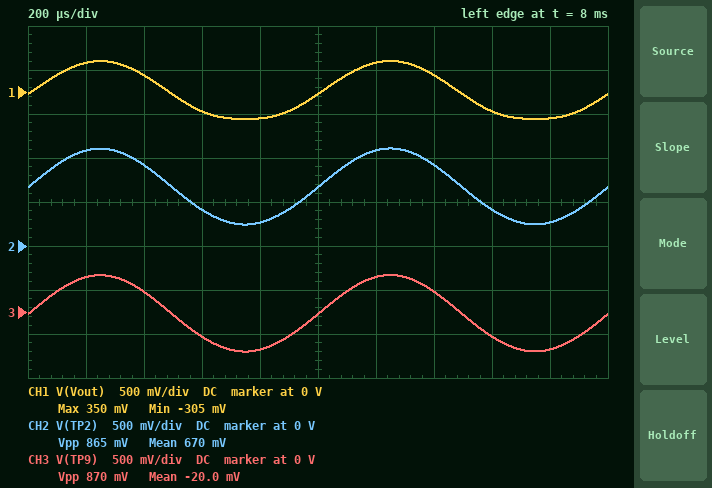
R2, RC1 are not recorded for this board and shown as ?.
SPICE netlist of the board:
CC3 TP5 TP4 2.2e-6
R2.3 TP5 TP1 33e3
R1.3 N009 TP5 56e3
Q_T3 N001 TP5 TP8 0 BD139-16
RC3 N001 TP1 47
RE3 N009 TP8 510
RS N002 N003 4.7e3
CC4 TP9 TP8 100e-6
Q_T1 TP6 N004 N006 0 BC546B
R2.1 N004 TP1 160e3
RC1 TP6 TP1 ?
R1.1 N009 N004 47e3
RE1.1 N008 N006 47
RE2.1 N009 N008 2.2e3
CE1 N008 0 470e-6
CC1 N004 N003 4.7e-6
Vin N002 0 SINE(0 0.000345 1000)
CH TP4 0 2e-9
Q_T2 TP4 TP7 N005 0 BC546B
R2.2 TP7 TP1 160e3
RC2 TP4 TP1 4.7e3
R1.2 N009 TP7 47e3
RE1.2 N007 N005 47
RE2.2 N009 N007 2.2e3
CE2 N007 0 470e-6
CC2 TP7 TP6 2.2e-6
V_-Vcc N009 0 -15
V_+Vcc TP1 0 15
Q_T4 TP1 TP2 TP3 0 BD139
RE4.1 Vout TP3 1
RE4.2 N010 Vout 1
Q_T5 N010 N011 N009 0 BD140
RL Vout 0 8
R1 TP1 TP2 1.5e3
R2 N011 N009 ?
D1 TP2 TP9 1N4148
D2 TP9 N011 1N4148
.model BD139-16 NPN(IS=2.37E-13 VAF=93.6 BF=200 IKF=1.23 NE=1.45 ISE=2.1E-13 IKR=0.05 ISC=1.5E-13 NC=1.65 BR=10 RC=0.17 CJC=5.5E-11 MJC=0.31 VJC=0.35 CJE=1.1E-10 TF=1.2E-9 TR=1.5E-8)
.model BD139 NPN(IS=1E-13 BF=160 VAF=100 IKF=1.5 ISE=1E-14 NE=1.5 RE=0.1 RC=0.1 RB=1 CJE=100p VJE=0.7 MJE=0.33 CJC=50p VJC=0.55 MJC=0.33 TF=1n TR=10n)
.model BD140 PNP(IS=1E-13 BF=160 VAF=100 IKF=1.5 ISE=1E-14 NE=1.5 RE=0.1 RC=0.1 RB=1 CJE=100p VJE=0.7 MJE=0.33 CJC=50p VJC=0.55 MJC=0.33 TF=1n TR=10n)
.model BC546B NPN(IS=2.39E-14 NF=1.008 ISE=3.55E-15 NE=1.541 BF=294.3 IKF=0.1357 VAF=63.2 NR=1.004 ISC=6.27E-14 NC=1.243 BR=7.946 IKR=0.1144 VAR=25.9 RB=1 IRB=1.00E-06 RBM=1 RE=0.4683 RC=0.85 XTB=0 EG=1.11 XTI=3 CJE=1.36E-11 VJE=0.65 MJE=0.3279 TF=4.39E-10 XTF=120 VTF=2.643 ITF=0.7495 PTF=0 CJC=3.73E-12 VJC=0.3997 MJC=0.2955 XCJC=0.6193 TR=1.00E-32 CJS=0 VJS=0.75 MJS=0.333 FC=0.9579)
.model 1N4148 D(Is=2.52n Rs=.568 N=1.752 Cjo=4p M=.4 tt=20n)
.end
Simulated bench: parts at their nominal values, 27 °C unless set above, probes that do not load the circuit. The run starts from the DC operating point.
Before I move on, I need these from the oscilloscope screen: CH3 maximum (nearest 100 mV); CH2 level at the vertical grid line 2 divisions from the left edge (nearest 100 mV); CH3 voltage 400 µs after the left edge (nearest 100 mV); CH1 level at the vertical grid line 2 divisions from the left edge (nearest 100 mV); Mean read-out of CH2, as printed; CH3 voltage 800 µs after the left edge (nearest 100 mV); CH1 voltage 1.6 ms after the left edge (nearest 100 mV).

400 mV
900 mV
200 mV
200 mV
670 mV
-400 mV
-200 mV
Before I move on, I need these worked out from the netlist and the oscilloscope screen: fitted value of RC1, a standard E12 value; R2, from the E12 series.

2.7 kΩ
680 Ω
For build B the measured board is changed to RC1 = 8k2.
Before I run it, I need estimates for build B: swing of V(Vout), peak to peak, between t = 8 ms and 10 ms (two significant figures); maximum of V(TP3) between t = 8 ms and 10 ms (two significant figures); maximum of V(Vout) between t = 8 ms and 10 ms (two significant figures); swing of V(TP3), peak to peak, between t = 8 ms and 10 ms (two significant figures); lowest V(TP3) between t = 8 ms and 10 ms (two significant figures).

1.1 V
830 mV
740 mV
1.2 V
-330 mV
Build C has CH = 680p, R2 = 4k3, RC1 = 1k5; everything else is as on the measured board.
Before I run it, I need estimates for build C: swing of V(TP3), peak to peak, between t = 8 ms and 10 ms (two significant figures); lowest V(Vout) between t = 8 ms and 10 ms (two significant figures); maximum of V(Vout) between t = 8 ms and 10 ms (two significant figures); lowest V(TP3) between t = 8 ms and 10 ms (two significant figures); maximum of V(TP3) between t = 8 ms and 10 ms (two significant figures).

670 mV
2.9 V
3.5 V
3.3 V
4.0 V
